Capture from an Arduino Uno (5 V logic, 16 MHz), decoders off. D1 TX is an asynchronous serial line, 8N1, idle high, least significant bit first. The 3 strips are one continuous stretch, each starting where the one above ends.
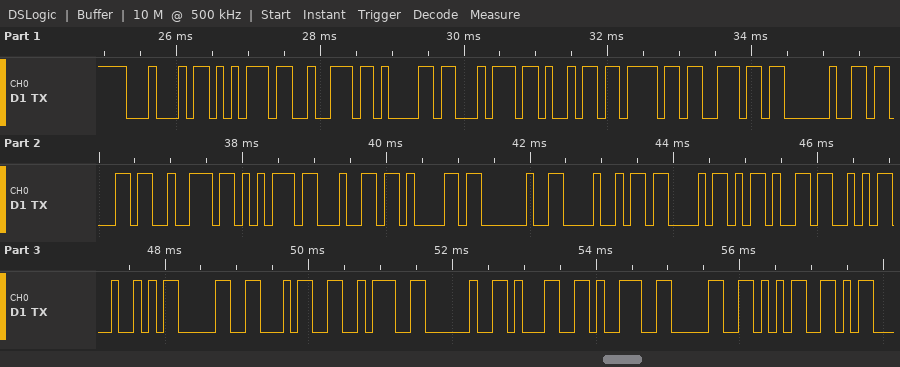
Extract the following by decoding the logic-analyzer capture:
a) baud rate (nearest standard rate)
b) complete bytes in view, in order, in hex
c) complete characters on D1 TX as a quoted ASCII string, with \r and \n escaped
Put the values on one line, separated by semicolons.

9600 baud; 44 75 72 61 74 69 6F 6E 20 63 72 75 64 61 20 48 43 2D 53 52 30 34 3A 20 31 39 30 35; "Duration cruda HC-SR04: 1905"
